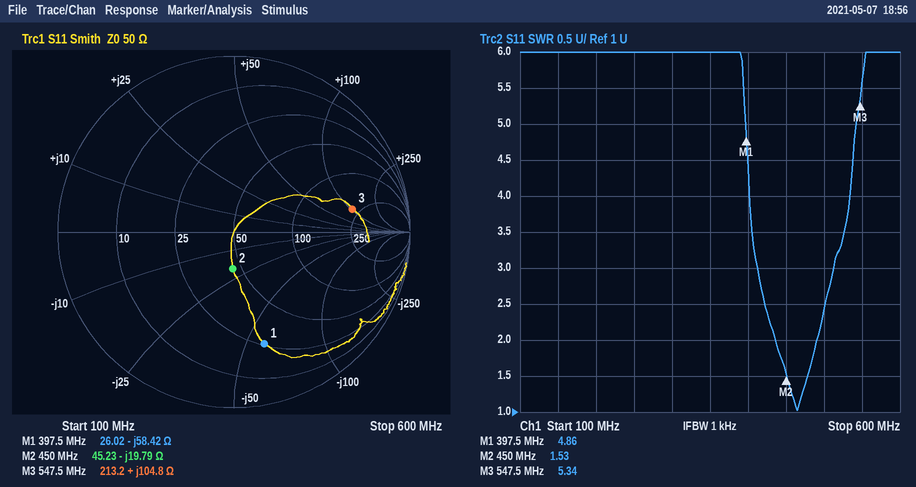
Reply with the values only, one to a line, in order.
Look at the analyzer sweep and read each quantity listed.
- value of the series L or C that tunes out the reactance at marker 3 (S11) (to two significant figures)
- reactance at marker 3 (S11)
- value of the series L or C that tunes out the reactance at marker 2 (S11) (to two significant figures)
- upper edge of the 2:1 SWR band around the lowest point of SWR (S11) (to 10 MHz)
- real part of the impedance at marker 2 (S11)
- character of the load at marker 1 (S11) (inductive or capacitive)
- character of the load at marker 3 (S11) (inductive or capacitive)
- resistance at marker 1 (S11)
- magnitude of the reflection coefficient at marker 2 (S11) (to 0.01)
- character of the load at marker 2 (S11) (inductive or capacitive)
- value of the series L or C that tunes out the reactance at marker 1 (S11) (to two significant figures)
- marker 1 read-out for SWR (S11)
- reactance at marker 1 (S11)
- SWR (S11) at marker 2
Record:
2.8 pF
+104.8 Ω
7.0 nH
490 MHz
45.23 Ω
capacitive
inductive
26.02 Ω
0.21
capacitive
23 nH
4.86
-58.42 Ω
1.53
